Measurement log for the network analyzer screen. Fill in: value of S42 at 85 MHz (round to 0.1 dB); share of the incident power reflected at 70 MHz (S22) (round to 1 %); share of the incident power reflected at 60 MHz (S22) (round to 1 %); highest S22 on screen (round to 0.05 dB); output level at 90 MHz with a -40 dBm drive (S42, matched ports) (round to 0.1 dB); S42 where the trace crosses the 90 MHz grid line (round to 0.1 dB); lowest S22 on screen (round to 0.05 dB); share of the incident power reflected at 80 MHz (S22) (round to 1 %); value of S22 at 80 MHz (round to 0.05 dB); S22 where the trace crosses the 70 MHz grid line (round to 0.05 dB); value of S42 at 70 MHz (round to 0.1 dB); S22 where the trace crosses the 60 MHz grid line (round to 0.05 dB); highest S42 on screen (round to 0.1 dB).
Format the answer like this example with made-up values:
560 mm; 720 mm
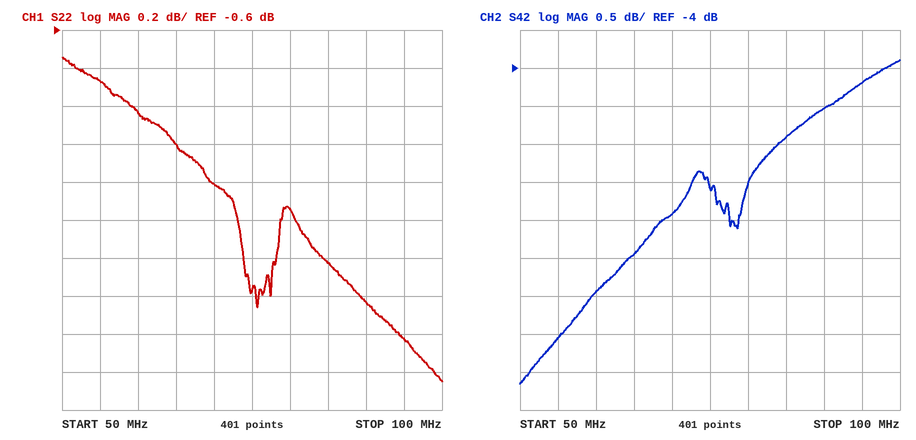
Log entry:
-4.9 dB; 72 %; 79 %; -0.75 dB; -44.5 dBm; -4.5 dB; -2.45 dB; 70 %; -1.55 dB; -1.40 dB; -5.9 dB; -1.05 dB; -3.9 dB
